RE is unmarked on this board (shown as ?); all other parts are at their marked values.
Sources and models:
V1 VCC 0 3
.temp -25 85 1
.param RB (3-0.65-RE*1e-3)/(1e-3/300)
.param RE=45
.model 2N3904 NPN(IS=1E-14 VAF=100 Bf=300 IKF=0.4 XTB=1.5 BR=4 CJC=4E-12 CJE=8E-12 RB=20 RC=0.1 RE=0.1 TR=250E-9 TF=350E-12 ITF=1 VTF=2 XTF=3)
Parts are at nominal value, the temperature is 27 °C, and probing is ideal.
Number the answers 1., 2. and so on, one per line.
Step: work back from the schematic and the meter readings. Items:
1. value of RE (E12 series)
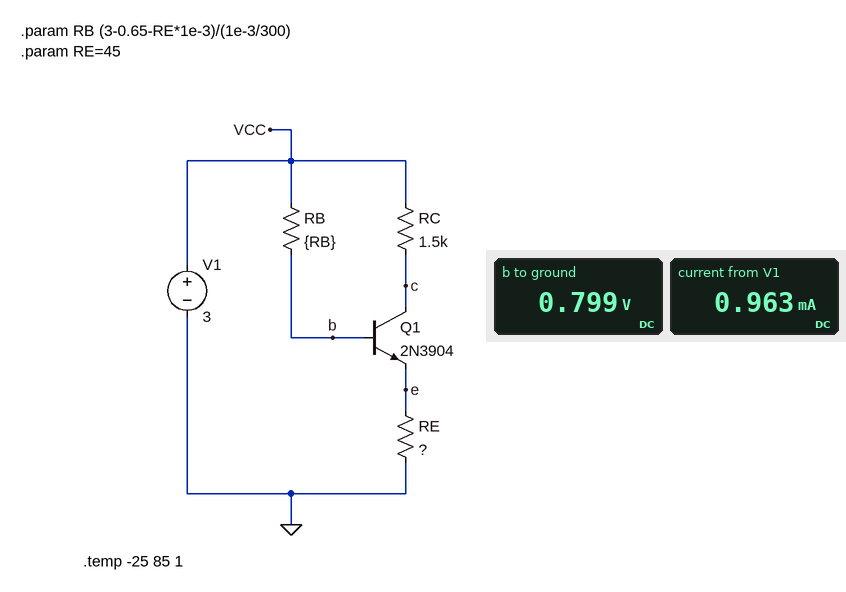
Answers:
1. 150 Ω
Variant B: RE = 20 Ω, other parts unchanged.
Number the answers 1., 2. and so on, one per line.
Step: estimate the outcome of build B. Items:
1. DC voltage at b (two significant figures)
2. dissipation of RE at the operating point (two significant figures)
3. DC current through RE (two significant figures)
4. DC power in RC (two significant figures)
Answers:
1. 680 mV
2. 21 µW
3. 1.0 mA
4. 1.5 mW
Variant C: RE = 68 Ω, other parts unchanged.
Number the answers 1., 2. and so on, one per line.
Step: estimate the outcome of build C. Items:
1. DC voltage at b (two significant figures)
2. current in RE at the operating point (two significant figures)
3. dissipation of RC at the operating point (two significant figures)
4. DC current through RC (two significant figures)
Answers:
1. 720 mV
2. 1.0 mA
3. 1.5 mW
4. 990 µA
